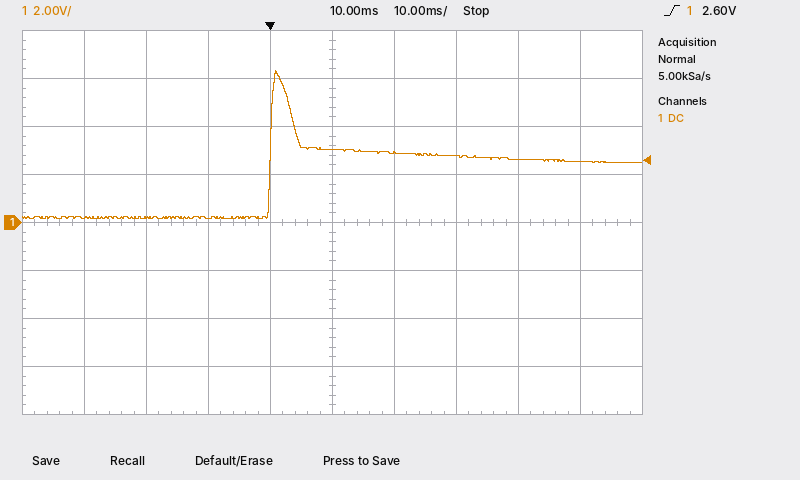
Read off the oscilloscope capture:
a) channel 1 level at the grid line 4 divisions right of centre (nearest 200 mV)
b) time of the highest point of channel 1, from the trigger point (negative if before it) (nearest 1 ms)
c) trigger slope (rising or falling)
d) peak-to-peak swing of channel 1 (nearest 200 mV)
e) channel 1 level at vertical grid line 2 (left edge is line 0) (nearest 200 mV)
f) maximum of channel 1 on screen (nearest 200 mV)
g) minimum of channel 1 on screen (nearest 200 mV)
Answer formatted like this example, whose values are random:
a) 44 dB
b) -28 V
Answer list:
a) 2.6 V
b) +1 ms
c) rising
d) 6.2 V
e) 200 mV
f) 6.4 V
g) 200 mV
